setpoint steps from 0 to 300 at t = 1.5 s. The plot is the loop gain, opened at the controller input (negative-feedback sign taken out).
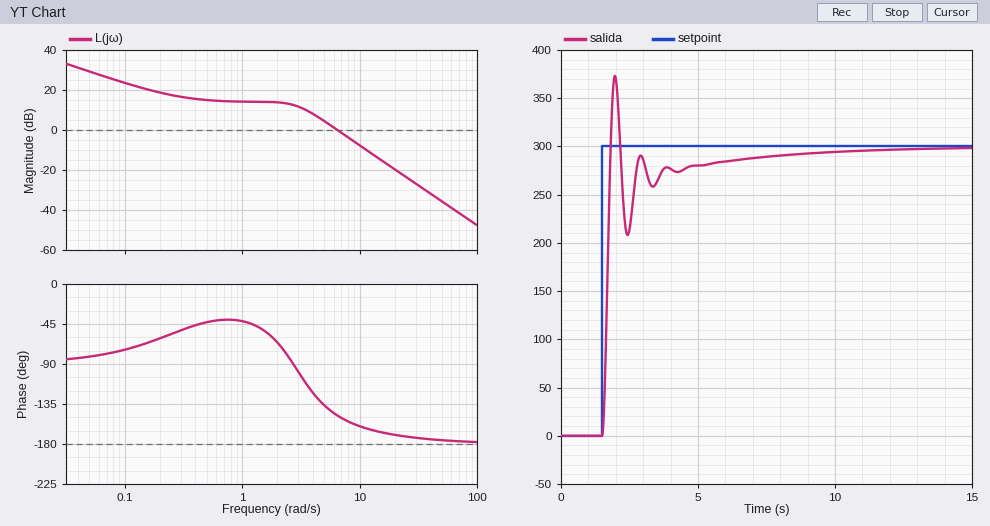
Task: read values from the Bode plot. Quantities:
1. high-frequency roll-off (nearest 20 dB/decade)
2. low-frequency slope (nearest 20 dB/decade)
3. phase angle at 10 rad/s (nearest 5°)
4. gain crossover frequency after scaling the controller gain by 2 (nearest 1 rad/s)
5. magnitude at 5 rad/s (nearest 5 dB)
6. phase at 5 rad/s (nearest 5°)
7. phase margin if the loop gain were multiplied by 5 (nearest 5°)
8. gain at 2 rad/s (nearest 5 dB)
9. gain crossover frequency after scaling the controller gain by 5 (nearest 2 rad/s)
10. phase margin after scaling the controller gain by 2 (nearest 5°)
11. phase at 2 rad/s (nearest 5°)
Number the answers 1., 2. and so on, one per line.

1. -40 dB/decade
2. -20 dB/decade
3. -160°
4. 9 rad/s
5. 5 dB
6. -135°
7. 15°
8. 15 dB
9. 14 rad/s
10. 20°
11. -65°
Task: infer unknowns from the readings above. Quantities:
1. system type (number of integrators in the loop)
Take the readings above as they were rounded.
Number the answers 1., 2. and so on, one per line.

1. 1
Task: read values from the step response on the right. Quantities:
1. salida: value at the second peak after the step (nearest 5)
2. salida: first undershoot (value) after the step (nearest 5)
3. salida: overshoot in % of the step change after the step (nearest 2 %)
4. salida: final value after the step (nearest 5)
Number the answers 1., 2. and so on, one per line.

1. 290
2. 210
3. 24 %
4. 300
